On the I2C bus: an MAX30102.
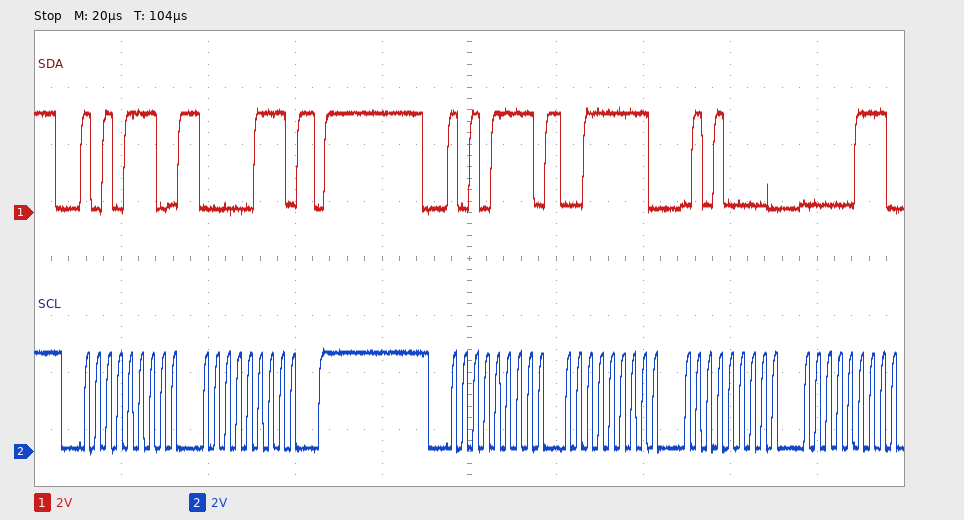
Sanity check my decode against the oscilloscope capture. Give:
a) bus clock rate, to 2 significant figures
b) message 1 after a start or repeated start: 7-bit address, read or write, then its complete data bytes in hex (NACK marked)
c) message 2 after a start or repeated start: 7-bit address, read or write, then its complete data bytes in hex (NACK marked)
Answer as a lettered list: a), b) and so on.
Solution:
a) 400 kHz
b) 0x57 write: 07
c) 0x57 read: 3F 50 07
